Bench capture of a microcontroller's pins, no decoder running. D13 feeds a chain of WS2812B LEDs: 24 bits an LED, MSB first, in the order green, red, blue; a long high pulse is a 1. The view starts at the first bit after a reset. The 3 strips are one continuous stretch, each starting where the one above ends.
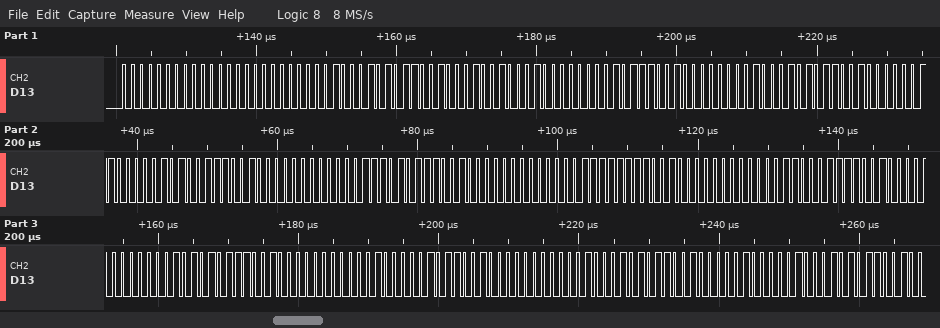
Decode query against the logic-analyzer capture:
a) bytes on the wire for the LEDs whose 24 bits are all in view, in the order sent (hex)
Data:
00 00 00 8A C8 91 00 B9 00 8A C8 18 29 C8 00 75 C8 00 3F C8 00 63 C8 00 55 C8 00 82 C8 00 8A C8 20
